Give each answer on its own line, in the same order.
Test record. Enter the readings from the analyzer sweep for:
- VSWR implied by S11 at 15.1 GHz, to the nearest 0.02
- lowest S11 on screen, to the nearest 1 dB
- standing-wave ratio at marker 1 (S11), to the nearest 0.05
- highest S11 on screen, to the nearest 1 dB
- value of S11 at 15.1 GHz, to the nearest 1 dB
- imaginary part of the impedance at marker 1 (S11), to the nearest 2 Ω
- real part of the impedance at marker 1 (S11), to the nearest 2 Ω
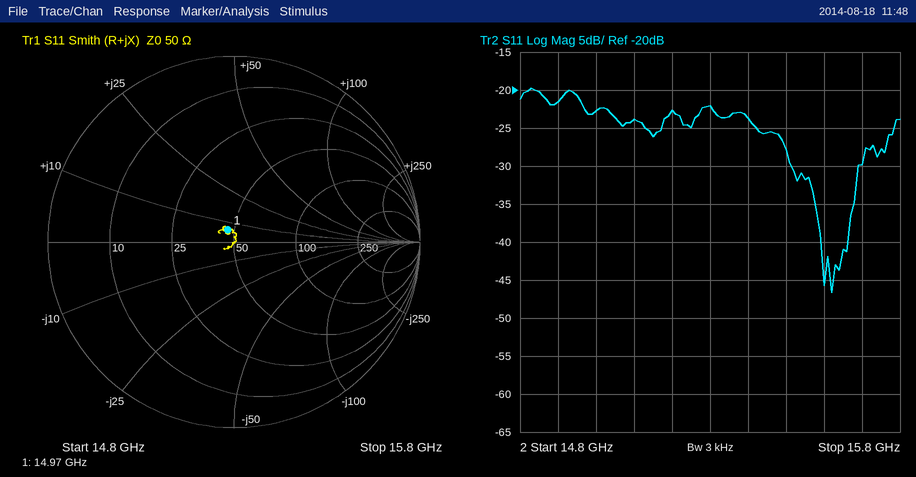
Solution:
1.14
-47 dB
1.15
-20 dB
-24 dB
+6 Ω
46 Ω
